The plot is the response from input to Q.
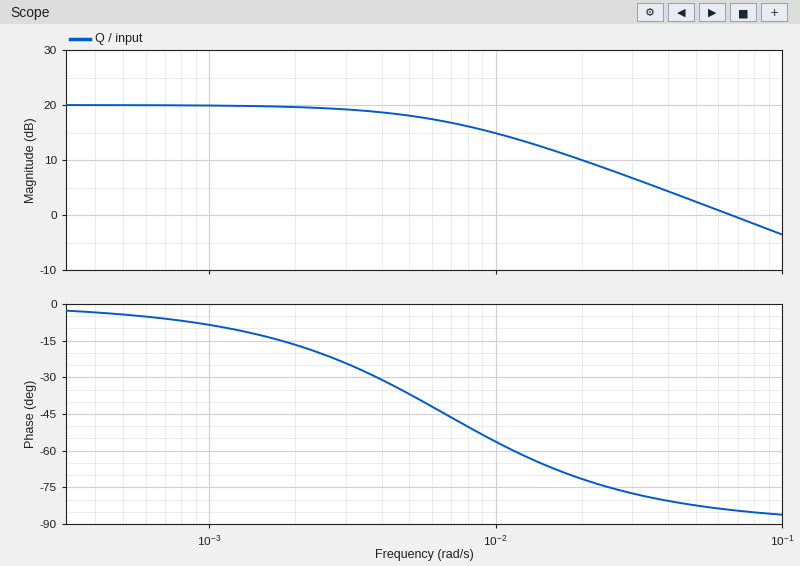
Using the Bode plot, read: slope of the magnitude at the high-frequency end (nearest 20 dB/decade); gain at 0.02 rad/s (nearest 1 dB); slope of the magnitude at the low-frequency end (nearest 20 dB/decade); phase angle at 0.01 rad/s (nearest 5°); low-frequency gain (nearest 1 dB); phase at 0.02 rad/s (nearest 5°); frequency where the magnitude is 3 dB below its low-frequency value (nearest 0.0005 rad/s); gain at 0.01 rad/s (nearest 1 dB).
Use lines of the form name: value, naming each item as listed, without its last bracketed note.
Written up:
slope of the magnitude at the high-frequency end: -20 dB/decade
gain at 0.02 rad/s: 10 dB
slope of the magnitude at the low-frequency end: 0 dB/decade
phase angle at 0.01 rad/s: -55°
low-frequency gain: 20 dB
phase at 0.02 rad/s: -70°
frequency where the magnitude is 3 dB below its low-frequency value: 0.0065 rad/s
gain at 0.01 rad/s: 15 dB
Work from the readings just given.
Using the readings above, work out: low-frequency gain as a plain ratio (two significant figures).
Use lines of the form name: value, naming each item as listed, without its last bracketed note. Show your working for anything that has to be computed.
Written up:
low-frequency gain as a plain ratio: 10^(20 / 20) = 10
